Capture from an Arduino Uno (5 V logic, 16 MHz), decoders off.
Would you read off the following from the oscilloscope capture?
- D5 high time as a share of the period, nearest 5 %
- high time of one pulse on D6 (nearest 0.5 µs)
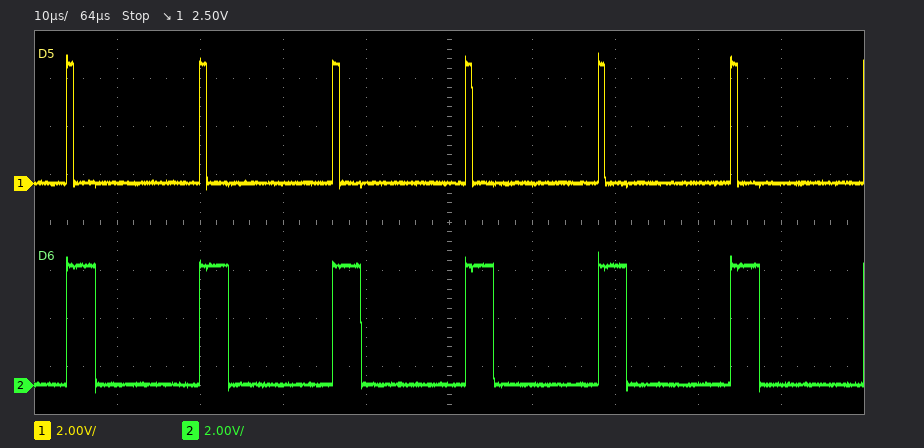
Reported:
5 %
3.5 µs
